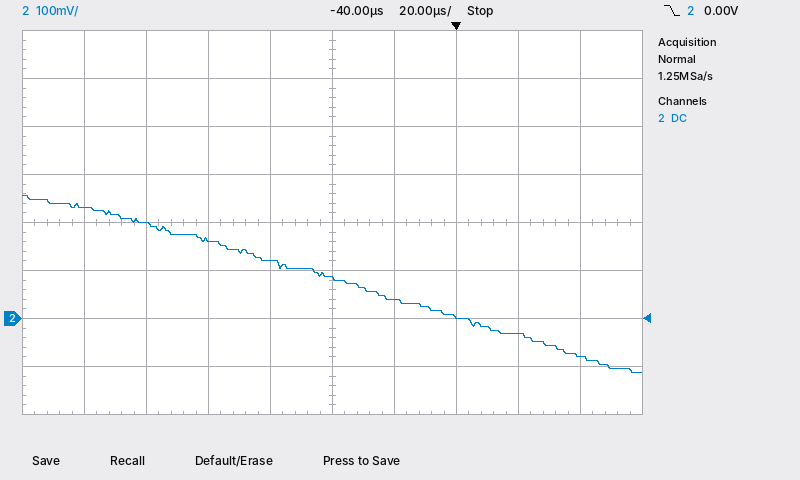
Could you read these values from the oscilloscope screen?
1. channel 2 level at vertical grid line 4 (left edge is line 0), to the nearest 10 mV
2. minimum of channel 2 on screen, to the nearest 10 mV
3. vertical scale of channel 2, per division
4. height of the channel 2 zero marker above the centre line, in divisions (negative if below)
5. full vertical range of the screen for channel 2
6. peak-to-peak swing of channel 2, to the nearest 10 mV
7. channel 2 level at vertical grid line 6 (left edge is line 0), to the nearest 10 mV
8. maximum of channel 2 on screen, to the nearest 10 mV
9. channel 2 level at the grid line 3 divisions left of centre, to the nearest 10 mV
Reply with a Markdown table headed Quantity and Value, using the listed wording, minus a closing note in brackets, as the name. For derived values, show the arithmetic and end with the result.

| Quantity | Value |
|---|---|
| channel 2 level at vertical grid line 4 (left edge is line 0), to the nearest 10 mV | 120 mV |
| minimum of channel 2 on screen, to the nearest 10 mV | -110 mV |
| vertical scale of channel 2, per division | 100 mV |
| height of the channel 2 zero marker above the centre line, in divisions | -2.0 div |
| full vertical range of the screen for channel 2 | 800 mV |
| peak-to-peak swing of channel 2, to the nearest 10 mV | 260 mV − (-110 mV) = 370 mV |
| channel 2 level at vertical grid line 6 (left edge is line 0), to the nearest 10 mV | 40 mV |
| maximum of channel 2 on screen, to the nearest 10 mV | 260 mV |
| channel 2 level at the grid line 3 divisions left of centre, to the nearest 10 mV | 200 mV |
